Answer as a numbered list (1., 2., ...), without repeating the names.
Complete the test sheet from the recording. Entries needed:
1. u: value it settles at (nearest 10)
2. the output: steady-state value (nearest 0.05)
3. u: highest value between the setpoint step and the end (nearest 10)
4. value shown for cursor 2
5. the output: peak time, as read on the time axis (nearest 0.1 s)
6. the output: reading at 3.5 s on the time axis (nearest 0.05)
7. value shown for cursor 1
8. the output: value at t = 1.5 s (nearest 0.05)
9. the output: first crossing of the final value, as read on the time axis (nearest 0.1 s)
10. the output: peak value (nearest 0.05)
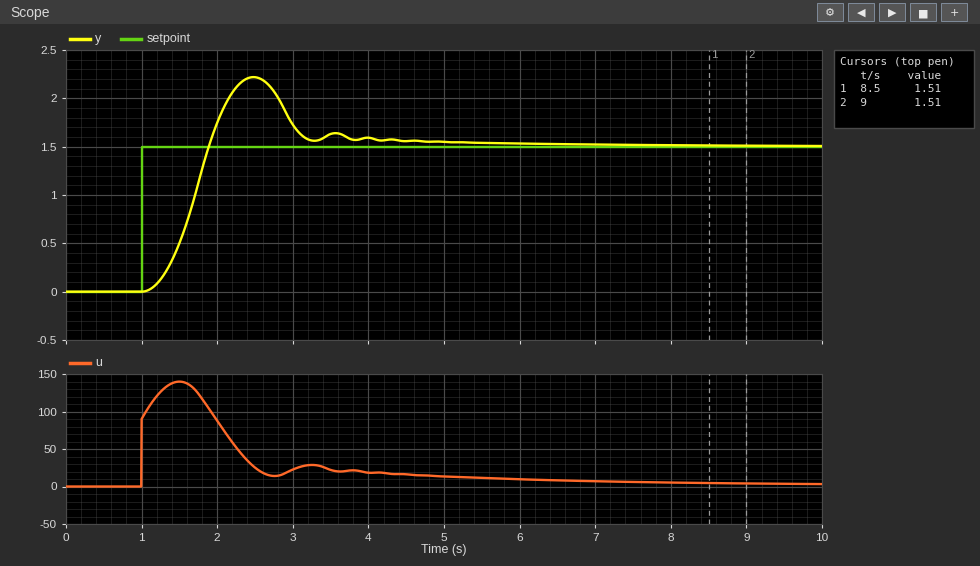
1. 0
2. 1.50
3. 140
4. 1.51
5. 2.5 s
6. 1.65
7. 1.51
8. 0.50
9. 1.9 s
10. 2.20
